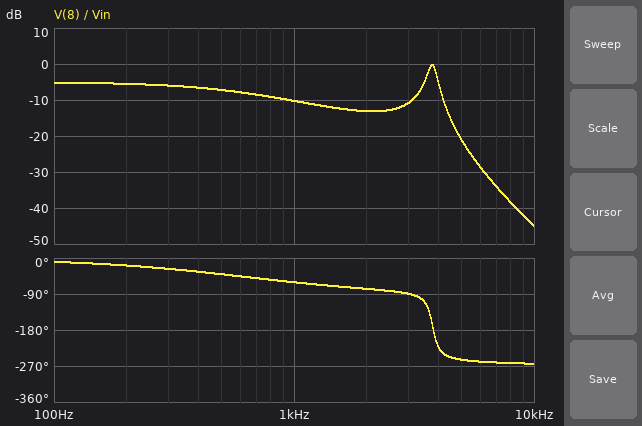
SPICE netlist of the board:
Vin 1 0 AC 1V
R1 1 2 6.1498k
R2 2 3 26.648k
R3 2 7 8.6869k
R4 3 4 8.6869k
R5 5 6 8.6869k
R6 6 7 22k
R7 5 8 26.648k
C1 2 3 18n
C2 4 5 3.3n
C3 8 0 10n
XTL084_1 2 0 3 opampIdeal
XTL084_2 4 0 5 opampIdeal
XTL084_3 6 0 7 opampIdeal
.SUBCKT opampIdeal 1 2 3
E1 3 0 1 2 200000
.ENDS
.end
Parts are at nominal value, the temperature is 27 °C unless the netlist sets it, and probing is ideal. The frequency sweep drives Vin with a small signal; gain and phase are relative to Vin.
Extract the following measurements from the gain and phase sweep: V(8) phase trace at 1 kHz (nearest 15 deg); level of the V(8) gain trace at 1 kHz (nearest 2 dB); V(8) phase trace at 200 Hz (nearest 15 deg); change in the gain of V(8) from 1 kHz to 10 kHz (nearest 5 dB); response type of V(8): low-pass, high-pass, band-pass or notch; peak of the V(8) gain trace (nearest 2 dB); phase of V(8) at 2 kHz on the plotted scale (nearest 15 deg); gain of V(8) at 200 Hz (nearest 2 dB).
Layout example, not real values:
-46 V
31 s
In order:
-60 deg
-10 dB
-15 deg
-35 dB
low-pass
0 dB
-75 deg
-6 dB
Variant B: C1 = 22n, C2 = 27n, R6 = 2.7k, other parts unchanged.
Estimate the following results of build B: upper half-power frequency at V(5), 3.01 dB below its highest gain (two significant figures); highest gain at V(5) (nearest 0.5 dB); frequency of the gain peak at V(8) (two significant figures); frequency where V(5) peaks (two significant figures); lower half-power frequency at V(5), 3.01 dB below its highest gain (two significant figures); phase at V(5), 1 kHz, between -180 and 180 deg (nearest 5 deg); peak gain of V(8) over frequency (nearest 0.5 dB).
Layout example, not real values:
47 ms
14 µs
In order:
500 Hz
17.5 dB
360 Hz
370 Hz
180 Hz
-160 deg
16.0 dB
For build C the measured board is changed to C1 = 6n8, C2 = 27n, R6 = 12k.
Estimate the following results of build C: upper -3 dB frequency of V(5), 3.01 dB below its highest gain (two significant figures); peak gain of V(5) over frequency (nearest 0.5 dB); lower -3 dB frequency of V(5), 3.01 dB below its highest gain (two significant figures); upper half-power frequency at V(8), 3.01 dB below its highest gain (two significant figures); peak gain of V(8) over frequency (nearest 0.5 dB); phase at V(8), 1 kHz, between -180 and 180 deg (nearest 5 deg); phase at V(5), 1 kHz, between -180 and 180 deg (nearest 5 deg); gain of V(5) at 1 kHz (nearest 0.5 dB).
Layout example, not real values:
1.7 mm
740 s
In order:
1.9 kHz
5.5 dB
890 Hz
1.5 kHz
0 dB
-90 deg
-30 deg
3.5 dB
